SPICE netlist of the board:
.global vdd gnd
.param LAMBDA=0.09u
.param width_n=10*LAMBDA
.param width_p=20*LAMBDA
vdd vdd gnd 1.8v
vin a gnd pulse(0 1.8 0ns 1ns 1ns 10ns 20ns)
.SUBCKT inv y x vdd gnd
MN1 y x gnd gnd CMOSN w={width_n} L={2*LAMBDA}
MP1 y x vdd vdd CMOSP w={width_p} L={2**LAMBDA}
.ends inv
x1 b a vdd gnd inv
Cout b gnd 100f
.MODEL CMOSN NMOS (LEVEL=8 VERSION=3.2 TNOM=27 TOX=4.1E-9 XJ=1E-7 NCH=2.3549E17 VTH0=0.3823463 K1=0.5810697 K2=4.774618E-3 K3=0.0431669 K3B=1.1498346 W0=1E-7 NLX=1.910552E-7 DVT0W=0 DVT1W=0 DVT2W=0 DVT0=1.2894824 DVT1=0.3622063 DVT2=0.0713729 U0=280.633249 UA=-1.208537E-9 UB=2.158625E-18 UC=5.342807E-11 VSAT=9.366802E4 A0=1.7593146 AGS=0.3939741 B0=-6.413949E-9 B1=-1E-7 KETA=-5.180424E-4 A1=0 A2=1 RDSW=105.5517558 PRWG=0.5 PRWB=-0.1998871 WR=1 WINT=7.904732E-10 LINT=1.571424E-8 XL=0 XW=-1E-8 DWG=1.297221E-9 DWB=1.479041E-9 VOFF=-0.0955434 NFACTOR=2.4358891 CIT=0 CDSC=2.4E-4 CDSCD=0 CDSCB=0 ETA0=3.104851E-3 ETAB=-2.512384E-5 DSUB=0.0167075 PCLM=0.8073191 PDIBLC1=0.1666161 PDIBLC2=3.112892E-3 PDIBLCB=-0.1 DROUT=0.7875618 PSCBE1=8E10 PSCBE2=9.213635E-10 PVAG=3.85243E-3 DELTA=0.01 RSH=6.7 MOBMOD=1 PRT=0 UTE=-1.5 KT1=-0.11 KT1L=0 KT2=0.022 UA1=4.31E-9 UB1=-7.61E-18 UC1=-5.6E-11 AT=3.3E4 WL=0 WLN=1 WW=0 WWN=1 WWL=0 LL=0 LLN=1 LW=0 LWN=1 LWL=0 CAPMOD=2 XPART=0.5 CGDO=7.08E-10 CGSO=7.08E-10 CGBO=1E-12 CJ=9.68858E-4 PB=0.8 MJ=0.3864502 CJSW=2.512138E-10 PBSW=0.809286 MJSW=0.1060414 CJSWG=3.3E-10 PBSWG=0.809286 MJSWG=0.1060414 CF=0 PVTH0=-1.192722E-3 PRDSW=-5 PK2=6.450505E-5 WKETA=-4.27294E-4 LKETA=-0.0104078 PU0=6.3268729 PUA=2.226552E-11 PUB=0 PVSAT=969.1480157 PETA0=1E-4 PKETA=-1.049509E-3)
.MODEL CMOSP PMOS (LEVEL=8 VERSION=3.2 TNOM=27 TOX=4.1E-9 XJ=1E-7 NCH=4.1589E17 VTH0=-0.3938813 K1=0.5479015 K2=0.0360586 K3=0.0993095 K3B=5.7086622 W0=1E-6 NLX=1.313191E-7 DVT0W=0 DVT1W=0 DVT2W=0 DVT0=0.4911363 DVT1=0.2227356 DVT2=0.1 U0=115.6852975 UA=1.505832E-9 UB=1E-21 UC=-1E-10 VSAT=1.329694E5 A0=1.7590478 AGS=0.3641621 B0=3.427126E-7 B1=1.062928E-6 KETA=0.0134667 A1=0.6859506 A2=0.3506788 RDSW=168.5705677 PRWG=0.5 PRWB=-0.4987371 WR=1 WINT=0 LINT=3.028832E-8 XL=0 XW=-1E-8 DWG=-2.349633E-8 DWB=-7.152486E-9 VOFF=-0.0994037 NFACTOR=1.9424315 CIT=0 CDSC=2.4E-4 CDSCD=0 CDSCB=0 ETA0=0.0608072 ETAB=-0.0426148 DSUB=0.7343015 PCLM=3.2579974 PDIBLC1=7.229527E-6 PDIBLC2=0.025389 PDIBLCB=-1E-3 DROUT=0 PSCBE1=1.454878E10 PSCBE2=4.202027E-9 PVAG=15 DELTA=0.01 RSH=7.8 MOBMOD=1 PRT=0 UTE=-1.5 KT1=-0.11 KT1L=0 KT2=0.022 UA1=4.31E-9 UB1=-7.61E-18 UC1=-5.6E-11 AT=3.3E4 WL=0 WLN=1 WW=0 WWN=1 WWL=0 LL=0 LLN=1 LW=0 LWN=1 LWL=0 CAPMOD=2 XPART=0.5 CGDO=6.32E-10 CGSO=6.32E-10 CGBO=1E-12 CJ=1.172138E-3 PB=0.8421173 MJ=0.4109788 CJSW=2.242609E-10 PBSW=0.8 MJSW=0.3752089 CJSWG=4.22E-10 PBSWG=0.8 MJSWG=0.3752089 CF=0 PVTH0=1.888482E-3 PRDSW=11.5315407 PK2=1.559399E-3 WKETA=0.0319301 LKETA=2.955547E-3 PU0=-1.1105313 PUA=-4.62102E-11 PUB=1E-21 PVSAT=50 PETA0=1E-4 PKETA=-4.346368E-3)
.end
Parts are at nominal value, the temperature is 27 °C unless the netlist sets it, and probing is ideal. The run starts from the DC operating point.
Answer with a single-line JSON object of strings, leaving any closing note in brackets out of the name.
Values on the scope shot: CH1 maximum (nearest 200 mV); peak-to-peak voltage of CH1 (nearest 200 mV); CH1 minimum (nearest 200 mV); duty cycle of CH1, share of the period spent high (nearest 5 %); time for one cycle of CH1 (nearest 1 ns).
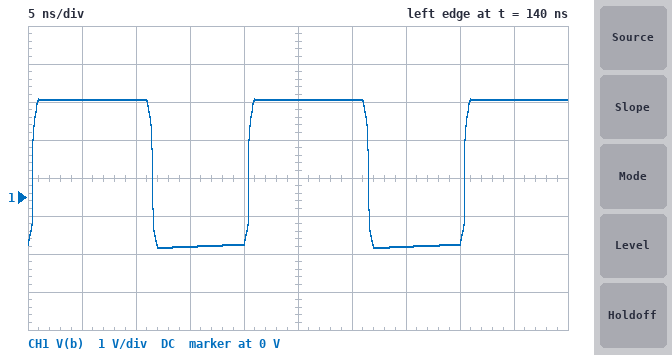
{"CH1 maximum": "2.6 V", "peak-to-peak voltage of CH1": "4.0 V", "CH1 minimum": "-1.4 V", "duty cycle of CH1, share of the period spent high": "55 %", "time for one cycle of CH1": "20 ns"}
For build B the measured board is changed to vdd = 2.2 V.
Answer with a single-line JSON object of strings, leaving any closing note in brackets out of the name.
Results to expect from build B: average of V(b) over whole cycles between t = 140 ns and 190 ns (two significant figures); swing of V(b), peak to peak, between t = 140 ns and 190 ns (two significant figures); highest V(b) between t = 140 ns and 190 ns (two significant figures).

{"average of V(b) over whole cycles between t = 140 ns and 190 ns": "1.1 V", "swing of V(b), peak to peak, between t = 140 ns and 190 ns": "4.2 V", "highest V(b) between t = 140 ns and 190 ns": "3.0 V"}
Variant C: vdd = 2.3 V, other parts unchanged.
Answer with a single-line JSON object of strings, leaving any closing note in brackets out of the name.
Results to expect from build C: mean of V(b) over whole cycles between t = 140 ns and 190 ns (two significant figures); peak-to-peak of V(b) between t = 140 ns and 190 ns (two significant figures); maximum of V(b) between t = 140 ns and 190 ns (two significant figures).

{"mean of V(b) over whole cycles between t = 140 ns and 190 ns": "1.2 V", "peak-to-peak of V(b) between t = 140 ns and 190 ns": "4.3 V", "maximum of V(b) between t = 140 ns and 190 ns": "3.1 V"}
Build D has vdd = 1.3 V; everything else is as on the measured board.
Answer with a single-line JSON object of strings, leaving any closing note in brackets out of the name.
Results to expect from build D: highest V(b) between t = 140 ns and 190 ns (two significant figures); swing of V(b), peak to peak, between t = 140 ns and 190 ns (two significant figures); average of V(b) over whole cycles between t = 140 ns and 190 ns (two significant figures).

{"highest V(b) between t = 140 ns and 190 ns": "2.1 V", "swing of V(b), peak to peak, between t = 140 ns and 190 ns": "3.5 V", "average of V(b) over whole cycles between t = 140 ns and 190 ns": "540 mV"}
